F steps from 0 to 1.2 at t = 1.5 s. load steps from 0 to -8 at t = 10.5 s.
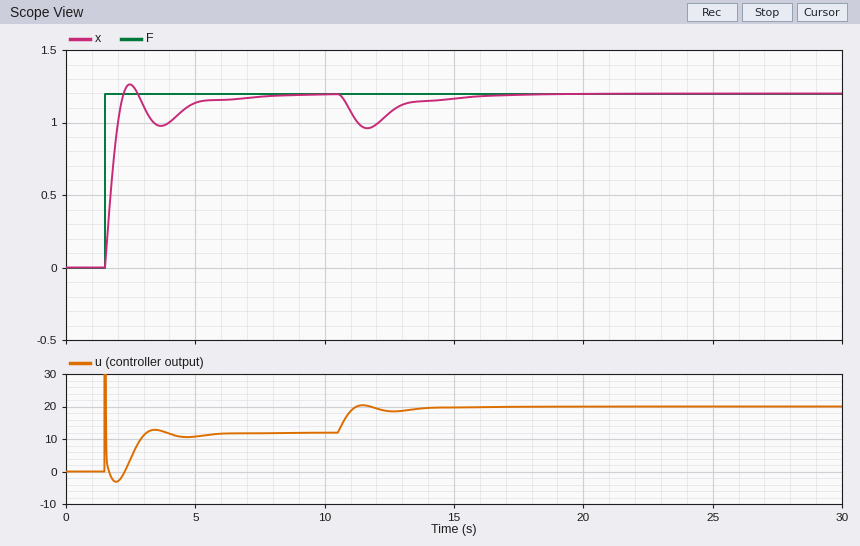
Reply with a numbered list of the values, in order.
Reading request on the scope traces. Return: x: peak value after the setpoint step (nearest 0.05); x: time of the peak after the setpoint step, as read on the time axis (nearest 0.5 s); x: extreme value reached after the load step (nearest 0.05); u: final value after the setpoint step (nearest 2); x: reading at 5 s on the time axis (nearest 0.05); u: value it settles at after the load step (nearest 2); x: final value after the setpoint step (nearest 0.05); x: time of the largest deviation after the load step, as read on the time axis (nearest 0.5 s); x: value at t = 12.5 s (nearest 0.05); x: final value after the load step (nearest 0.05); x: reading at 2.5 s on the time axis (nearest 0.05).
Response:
1. 1.25
2. 2.5 s
3. 0.95
4. 12
5. 1.15
6. 20
7. 1.20
8. 11.5 s
9. 1.05
10. 1.20
11. 1.25
